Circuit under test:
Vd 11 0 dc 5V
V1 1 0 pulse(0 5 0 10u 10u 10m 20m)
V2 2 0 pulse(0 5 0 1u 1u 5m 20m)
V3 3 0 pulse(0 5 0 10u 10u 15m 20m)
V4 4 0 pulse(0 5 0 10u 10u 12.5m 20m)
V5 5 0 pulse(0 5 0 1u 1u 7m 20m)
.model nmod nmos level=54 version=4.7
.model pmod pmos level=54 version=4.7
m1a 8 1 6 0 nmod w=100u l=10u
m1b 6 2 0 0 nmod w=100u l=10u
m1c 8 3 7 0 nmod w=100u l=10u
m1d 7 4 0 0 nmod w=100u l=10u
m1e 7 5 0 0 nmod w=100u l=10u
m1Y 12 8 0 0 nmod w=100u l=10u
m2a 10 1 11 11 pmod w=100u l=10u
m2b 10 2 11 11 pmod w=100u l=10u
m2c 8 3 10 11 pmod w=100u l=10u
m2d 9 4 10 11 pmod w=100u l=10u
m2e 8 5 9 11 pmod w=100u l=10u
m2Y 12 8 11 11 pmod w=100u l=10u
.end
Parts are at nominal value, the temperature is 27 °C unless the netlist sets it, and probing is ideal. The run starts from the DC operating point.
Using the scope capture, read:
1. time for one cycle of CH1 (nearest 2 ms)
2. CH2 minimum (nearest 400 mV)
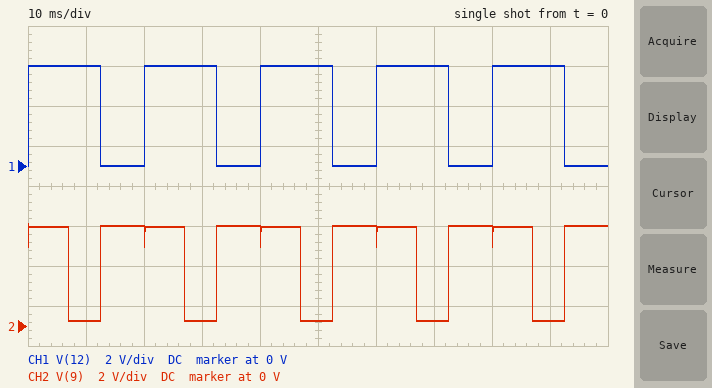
20 ms
400 mV
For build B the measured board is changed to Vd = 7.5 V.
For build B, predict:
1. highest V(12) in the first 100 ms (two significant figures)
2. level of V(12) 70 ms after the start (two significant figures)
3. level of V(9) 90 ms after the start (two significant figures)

7.5 V
7.1 V
2.2 V
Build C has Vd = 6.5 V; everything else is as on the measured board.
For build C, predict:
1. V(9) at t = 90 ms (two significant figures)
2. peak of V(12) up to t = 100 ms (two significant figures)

1.4 V
6.5 V
